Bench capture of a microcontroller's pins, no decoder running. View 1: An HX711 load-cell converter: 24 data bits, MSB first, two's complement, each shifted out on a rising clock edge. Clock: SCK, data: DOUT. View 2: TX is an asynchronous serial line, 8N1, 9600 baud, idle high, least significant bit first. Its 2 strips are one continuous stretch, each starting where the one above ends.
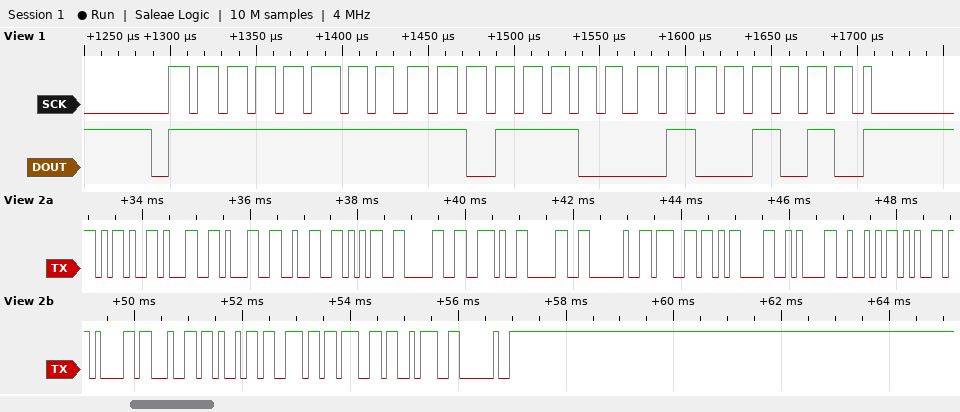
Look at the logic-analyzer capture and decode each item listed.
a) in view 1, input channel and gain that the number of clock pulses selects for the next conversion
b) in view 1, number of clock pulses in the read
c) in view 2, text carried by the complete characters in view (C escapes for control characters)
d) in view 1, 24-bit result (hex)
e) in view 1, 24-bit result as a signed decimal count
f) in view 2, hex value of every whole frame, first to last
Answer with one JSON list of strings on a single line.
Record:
["channel A, gain 128", "25", "\"-11250.0 g\\r\\nReading: \"", "0xFFDC4A", "-9142", "2D 31 31 32 35 30 2E 30 20 67 0D 0A 52 65 61 64 69 6E 67 3A 20"]
